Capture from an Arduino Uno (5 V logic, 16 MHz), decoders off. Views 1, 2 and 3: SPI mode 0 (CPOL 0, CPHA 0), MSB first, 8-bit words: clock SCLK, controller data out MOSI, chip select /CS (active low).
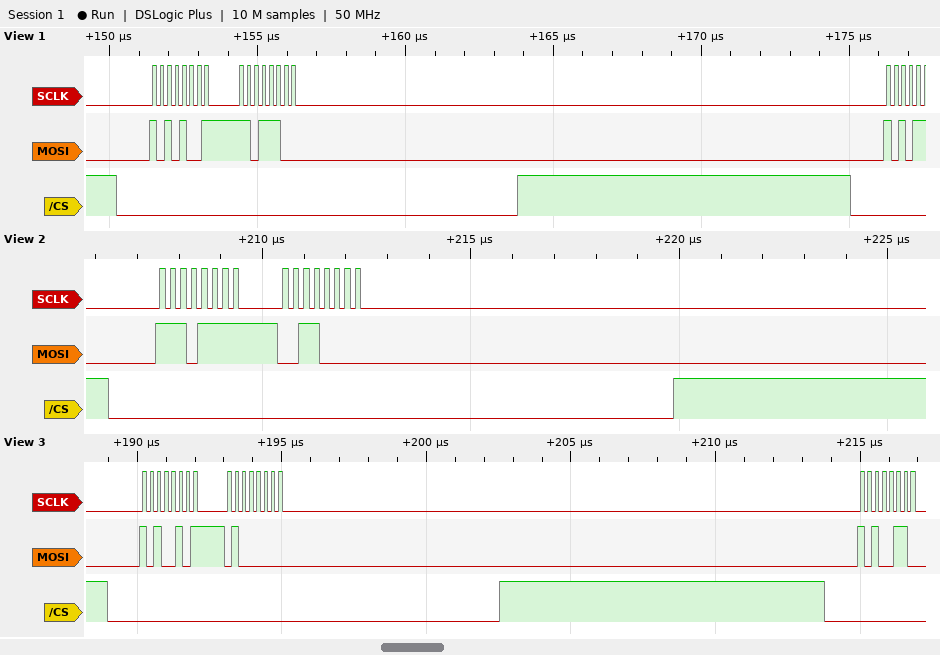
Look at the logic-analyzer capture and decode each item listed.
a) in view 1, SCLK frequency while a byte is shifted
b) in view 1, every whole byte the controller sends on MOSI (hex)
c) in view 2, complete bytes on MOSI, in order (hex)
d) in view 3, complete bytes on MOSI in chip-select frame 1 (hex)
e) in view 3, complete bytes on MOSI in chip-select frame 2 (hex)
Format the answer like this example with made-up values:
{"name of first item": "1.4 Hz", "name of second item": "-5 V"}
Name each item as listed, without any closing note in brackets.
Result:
{"in view 1, SCLK frequency while a byte is shifted": "4 MHz", "in view 1, every whole byte the controller sends on MOSI": "A9 DC", "in view 2, complete bytes on MOSI, in order": "EF 30", "in view 3, complete bytes on MOSI in chip-select frame 1": "A5 40", "in view 3, complete bytes on MOSI in chip-select frame 2": "A6"}
